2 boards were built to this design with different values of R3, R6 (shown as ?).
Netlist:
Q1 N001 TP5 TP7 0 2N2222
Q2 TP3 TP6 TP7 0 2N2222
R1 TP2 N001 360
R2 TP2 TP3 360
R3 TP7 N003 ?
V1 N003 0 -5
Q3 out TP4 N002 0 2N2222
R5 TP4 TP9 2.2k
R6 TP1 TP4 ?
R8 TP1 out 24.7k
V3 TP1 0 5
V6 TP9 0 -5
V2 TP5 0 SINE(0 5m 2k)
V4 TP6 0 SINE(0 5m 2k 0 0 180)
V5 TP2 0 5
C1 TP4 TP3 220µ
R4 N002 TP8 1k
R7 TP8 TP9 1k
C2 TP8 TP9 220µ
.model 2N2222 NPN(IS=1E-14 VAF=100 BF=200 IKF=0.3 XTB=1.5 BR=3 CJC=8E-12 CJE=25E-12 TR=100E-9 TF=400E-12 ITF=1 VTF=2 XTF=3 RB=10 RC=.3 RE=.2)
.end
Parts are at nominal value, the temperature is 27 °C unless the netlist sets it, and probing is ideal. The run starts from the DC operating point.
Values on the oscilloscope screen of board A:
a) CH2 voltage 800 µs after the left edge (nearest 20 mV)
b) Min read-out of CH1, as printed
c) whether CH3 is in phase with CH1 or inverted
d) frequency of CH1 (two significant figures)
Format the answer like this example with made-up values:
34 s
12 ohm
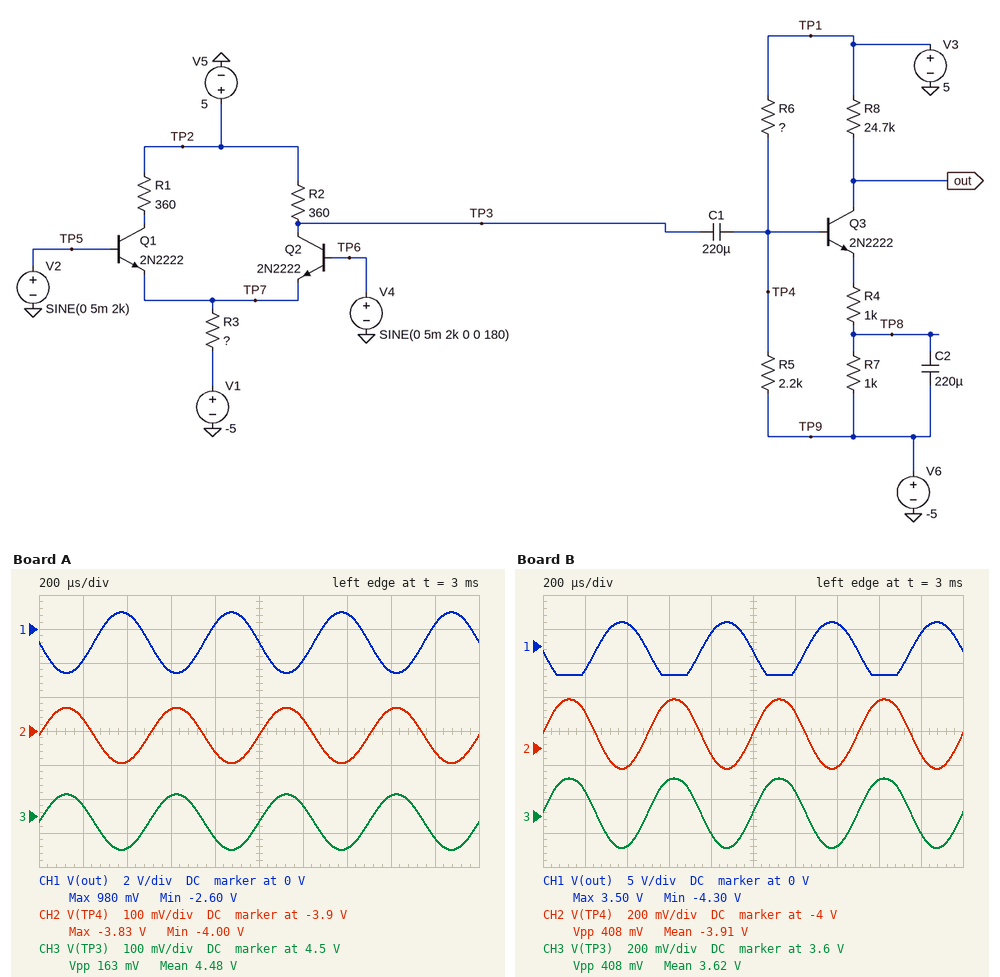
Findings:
-3.96 V
-2.60 V
inverted
2.0 kHz
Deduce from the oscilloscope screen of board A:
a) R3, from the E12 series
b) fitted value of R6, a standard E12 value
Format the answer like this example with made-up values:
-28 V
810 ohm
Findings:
1.5 kΩ
18 kΩ
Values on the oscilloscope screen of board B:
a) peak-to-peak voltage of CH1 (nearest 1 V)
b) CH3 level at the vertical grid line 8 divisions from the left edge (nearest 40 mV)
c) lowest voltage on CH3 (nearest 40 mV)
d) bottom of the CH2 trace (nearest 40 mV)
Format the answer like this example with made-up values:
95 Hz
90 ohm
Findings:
8 V
3.80 V
3.40 V
-4.12 V
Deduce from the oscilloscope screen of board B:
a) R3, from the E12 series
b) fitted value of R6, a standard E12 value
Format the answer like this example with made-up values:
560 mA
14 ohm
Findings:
560 Ω
18 kΩ
